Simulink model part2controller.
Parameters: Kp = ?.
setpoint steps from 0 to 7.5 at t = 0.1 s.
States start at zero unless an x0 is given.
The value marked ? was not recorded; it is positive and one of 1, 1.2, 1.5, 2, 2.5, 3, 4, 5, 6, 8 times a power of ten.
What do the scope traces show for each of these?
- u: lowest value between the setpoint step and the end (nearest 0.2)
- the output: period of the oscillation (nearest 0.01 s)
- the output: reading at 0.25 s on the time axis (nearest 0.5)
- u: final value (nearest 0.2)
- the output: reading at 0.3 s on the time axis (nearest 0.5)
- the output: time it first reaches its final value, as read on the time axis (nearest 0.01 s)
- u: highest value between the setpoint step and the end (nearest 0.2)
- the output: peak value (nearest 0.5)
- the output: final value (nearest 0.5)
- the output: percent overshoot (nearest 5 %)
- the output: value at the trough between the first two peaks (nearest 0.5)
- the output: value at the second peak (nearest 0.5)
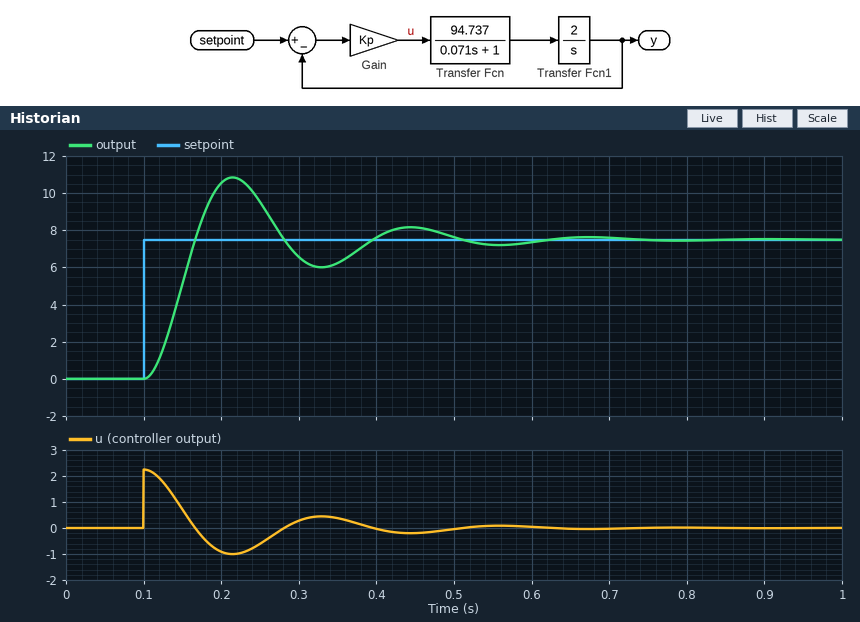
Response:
-1.0
0.23 s
9.5
0.0
6.5
0.17 s
2.2
11.0
7.5
45 %
6.0
8.0
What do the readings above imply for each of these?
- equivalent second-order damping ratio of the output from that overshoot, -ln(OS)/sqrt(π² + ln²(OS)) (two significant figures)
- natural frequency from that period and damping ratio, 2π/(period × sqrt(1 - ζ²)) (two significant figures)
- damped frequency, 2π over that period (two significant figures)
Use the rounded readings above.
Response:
0.25
28 rad/s
27 rad/s
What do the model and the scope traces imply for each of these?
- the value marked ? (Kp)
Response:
0.3
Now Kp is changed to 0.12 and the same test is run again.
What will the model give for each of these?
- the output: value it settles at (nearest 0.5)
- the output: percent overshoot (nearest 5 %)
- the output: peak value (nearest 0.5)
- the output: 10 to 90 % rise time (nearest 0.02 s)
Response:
7.5
25 %
9.5
0.08 s
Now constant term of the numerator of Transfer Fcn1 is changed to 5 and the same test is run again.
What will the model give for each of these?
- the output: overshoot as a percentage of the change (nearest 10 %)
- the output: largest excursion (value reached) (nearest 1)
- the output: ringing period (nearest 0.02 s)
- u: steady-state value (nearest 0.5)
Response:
60 %
12
0.14 s
0.0
